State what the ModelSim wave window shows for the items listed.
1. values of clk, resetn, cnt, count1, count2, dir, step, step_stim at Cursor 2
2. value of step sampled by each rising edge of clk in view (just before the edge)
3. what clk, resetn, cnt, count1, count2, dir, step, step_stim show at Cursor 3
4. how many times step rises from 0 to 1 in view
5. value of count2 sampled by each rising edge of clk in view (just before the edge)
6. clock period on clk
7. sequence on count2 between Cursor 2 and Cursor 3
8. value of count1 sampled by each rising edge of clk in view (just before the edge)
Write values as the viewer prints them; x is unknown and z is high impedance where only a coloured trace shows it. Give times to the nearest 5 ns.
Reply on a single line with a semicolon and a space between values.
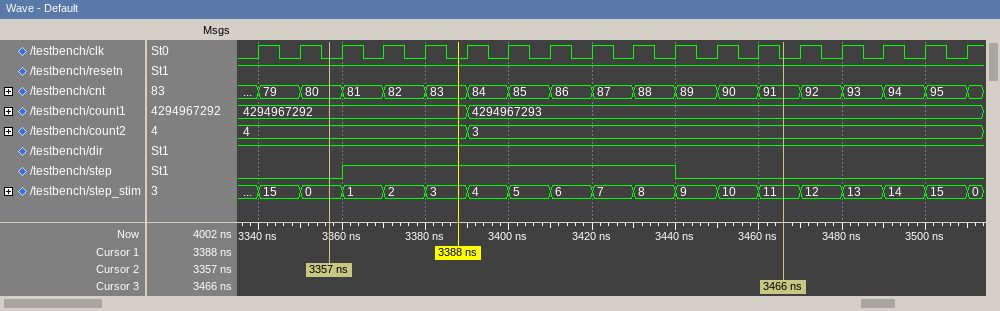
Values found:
clk=0, resetn=1, cnt=80, count1=4294967292, count2=4, dir=1, step=0, step_stim=0; 0 0 0 1 1 1 1 1 1 1 1 0 0 0 0 0 0 0; clk=0, resetn=1, cnt=91, count1=4294967293, count2=3, dir=1, step=0, step_stim=11; 1; 4, 4, 4, 4, 4, 4, 3, 3, 3, 3, 3, 3, 3, 3, 3, 3, 3, 3; 10 ns; 4, 3; 4294967292, 4294967292, 4294967292, 4294967292, 4294967292, 4294967292, 4294967293, 4294967293, 4294967293, 4294967293, 4294967293, 4294967293, 4294967293, 4294967293, 4294967293, 4294967293, 4294967293, 4294967293
